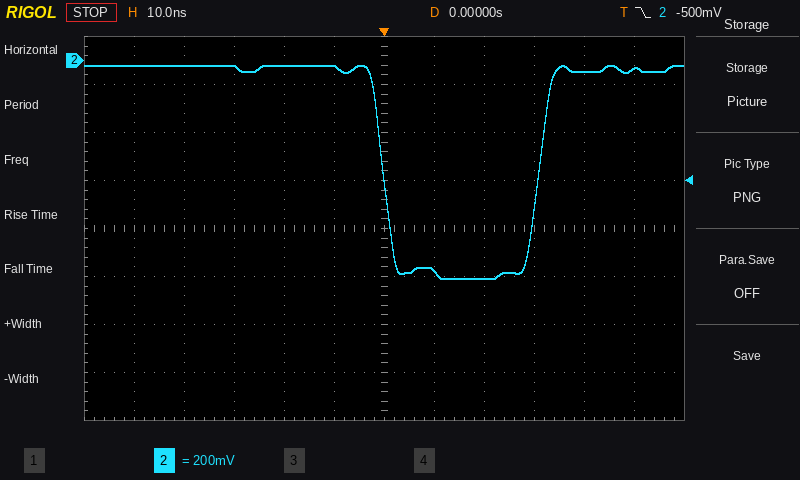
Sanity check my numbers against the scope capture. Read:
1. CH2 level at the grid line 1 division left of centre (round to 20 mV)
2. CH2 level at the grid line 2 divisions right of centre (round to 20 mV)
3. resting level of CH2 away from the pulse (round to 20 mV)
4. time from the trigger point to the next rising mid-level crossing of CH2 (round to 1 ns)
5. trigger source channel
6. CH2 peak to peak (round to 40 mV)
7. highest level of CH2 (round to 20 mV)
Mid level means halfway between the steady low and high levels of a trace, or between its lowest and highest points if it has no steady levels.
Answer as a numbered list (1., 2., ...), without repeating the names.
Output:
1. -20 mV
2. -900 mV
3. -20 mV
4. 31 ns
5. CH2
6. 880 mV
7. -20 mV
